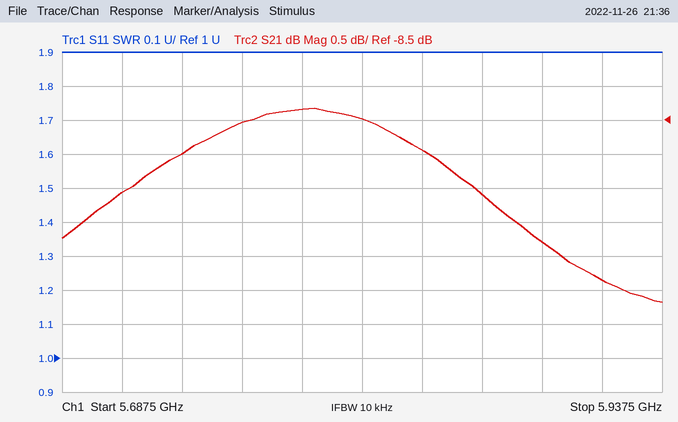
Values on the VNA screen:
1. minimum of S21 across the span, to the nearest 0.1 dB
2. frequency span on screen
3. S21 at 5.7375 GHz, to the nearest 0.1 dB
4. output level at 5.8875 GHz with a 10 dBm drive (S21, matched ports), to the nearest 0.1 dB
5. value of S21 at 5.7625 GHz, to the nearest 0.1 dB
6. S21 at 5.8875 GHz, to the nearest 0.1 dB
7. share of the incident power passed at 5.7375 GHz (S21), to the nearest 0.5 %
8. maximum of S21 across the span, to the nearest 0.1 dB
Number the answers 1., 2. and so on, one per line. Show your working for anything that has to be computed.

1. -11.2 dB
2. 250 MHz
3. -9.0 dB
4. 10 dBm + (-10.3 dB) = -0.3 dBm
5. -8.5 dB
6. -10.3 dB
7. 10^(-9/10) ≈ 12.6 %, so 12.5 % to the nearest 0.5 %
8. -8.3 dB
